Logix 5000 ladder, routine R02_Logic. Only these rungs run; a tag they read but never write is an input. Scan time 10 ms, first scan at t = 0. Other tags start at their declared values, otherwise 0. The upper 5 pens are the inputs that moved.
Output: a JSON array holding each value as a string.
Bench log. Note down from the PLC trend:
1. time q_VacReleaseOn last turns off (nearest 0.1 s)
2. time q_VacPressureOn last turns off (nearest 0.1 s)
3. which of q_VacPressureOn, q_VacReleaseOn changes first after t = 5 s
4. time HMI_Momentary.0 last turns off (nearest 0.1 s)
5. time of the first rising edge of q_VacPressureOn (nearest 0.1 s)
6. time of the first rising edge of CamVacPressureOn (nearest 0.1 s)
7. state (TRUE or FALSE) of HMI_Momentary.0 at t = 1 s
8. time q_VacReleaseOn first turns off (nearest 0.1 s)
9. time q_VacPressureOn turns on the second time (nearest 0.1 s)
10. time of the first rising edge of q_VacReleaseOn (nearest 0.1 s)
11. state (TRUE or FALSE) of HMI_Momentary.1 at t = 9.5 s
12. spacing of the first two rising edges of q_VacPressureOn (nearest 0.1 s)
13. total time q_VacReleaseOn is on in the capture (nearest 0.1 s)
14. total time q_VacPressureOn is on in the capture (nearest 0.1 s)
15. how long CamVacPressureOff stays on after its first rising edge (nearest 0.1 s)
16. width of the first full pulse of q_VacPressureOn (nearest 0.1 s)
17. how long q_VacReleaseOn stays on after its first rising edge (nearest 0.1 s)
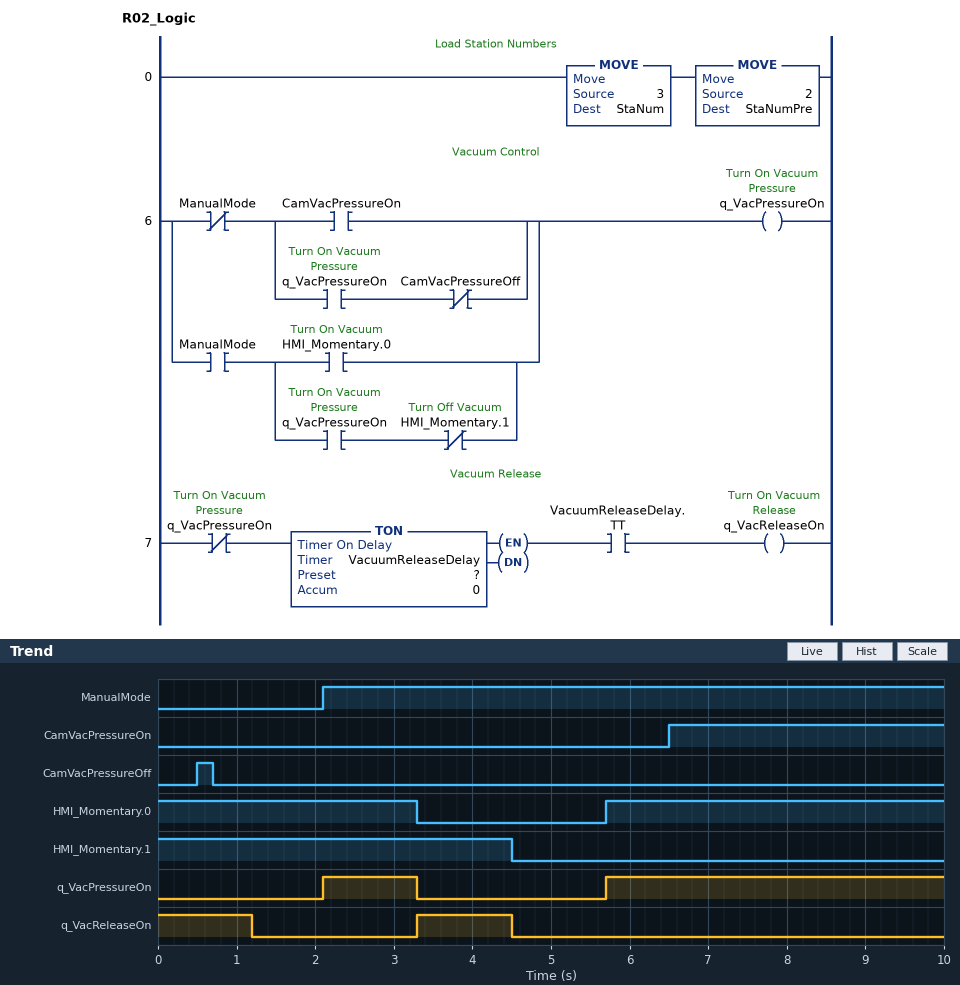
["4.5 s", "3.3 s", "q_VacPressureOn", "3.3 s", "2.1 s", "6.5 s", "TRUE", "1.2 s", "5.7 s", "3.3 s", "FALSE", "3.6 s", "2.4 s", "5.5 s", "0.2 s", "1.2 s", "1.2 s"]
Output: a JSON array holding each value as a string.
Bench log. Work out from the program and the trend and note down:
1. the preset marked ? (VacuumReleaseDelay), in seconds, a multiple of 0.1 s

["1.2 s"]
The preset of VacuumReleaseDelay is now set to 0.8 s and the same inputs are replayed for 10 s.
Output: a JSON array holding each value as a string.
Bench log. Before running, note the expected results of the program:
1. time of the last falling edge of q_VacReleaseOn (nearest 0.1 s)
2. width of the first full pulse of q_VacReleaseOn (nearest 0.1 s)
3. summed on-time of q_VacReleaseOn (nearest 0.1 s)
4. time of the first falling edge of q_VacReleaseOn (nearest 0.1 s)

["4.1 s", "0.8 s", "1.6 s", "0.8 s"]
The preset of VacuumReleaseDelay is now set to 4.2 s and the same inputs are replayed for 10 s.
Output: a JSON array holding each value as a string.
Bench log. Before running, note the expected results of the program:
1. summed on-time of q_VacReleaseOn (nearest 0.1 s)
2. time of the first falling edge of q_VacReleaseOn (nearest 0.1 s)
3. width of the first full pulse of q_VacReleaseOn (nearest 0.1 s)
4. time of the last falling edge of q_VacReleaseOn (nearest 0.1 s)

["4.5 s", "2.1 s", "2.4 s", "5.7 s"]
